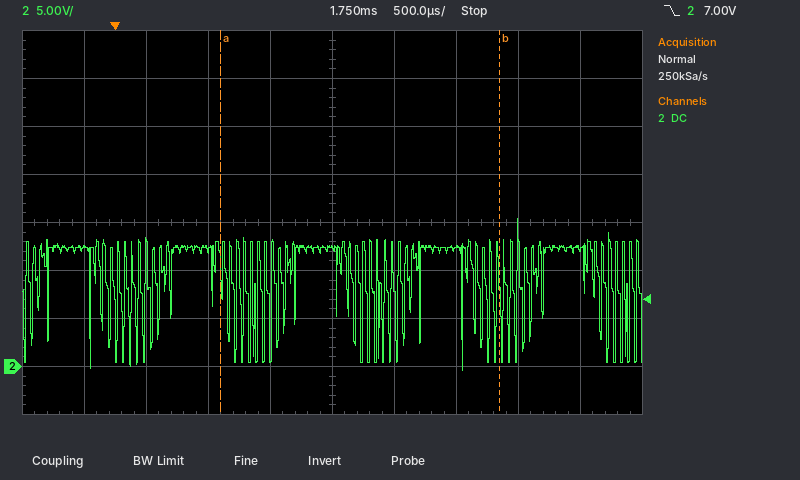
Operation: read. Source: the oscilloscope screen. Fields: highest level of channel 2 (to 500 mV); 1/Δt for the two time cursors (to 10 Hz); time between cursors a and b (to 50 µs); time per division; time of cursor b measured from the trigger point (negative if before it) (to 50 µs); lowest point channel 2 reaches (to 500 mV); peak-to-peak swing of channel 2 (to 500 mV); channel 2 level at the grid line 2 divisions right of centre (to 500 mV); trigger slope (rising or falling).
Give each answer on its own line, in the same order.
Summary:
15.5 V
440 Hz
2.25 ms
500 µs
+3.10 ms
-500 mV
16.0 V
12.5 V
falling
